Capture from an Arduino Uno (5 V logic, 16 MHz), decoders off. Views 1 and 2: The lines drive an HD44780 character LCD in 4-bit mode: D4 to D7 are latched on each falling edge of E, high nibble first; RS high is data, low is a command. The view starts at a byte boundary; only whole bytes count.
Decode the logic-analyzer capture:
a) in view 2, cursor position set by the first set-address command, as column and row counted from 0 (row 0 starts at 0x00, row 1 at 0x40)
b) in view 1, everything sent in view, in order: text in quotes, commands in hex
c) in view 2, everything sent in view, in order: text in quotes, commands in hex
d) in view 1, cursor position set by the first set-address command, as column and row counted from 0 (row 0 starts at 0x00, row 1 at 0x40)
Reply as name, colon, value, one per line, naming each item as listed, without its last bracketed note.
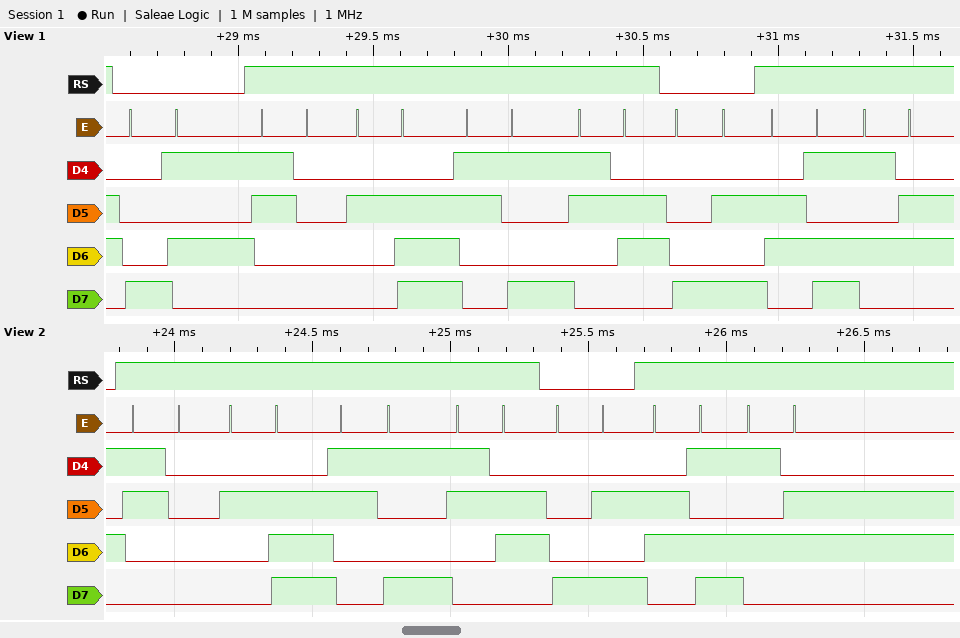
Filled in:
in view 2, cursor position set by the first set-address command, as column and row counted from 0: column 10, row 0
in view 1, everything sent in view, in order: text in quotes, commands in hex: 0x85 "0.96" 0x8A "mV"
in view 2, everything sent in view, in order: text in quotes, commands in hex: "0.96" 0x8A "mV"
in view 1, cursor position set by the first set-address command, as column and row counted from 0: column 5, row 0
